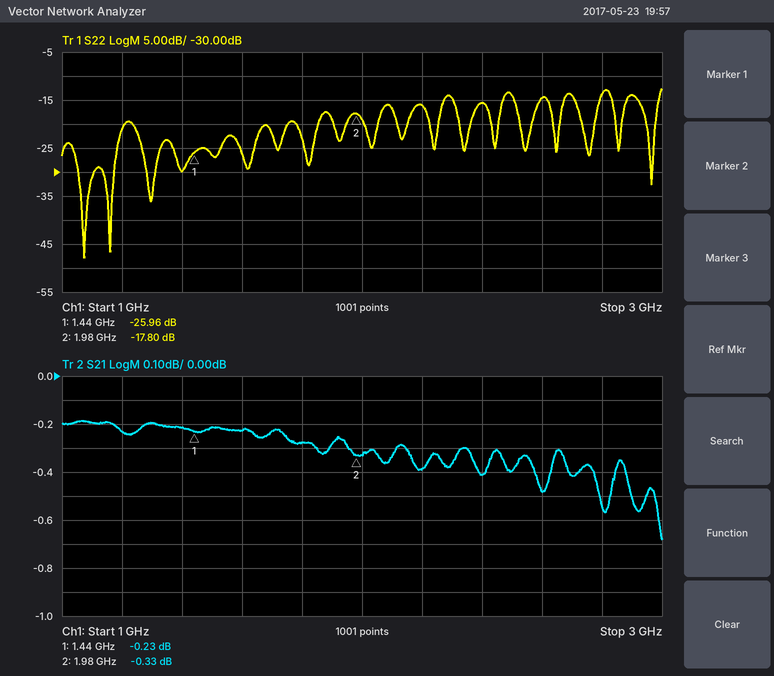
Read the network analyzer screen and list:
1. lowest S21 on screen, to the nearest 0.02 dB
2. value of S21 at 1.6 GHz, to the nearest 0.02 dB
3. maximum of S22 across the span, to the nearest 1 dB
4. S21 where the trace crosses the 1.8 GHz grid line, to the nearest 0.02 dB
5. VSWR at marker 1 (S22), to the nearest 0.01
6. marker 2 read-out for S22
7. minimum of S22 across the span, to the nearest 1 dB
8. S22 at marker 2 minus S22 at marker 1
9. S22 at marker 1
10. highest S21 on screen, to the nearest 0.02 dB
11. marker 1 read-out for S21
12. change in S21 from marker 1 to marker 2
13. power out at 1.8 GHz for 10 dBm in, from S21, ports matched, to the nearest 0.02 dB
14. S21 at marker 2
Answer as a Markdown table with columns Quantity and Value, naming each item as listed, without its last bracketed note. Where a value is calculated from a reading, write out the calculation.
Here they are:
| Quantity | Value |
|---|---|
| lowest S21 on screen, to the nearest 0.02 dB | -0.68 dB |
| value of S21 at 1.6 GHz, to the nearest 0.02 dB | -0.22 dB |
| maximum of S22 across the span, to the nearest 1 dB | -13 dB |
| S21 where the trace crosses the 1.8 GHz grid line, to the nearest 0.02 dB | -0.28 dB |
| VSWR at marker 1 (S22), to the nearest 0.01 | (1 + 0.0504)/(1 − 0.0504) ≈ 1.11 |
| marker 2 read-out for S22 | -17.80 dB |
| minimum of S22 across the span, to the nearest 1 dB | -48 dB |
| S22 at marker 2 minus S22 at marker 1 | -17.8 − (-25.96) = 8.16 dB |
| S22 at marker 1 | -25.96 dB |
| highest S21 on screen, to the nearest 0.02 dB | -0.18 dB |
| marker 1 read-out for S21 | -0.23 dB |
| change in S21 from marker 1 to marker 2 | -0.33 − (-0.23) = -0.10 dB |
| power out at 1.8 GHz for 10 dBm in, from S21, ports matched, to the nearest 0.02 dB | 10 dBm + (-0.28 dB) = 9.72 dBm |
| S21 at marker 2 | -0.33 dB |
